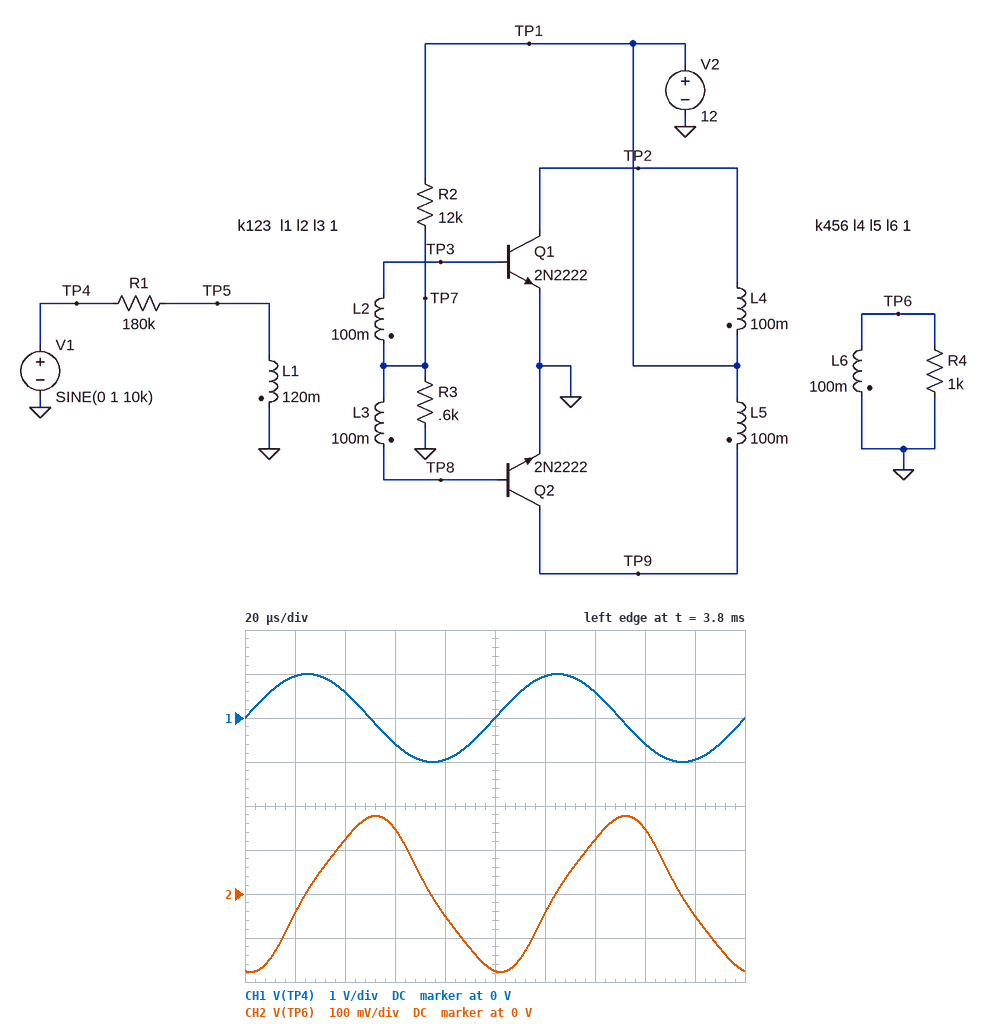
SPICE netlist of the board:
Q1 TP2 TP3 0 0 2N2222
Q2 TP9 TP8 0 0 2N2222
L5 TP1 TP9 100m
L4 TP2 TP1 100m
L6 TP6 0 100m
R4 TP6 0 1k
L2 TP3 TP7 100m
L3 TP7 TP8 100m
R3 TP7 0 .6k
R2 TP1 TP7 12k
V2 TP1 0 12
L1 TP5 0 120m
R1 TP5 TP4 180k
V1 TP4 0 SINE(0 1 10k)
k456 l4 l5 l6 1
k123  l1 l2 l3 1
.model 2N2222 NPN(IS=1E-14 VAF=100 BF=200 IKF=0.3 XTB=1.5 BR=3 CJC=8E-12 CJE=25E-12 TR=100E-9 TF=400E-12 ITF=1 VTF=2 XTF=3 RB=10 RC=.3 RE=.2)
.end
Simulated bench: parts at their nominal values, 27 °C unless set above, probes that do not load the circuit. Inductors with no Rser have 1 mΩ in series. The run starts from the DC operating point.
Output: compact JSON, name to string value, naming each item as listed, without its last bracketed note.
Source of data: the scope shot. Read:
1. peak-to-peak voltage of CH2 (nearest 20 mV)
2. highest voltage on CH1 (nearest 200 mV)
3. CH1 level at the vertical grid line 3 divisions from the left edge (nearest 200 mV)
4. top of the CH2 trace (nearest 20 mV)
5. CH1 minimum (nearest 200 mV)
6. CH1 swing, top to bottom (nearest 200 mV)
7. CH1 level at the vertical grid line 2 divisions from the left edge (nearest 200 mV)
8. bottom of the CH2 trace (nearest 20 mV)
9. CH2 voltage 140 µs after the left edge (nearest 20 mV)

{"peak-to-peak voltage of CH2": "360 mV", "highest voltage on CH1": "1.0 V", "CH1 level at the vertical grid line 3 divisions from the left edge": "-600 mV", "top of the CH2 trace": "180 mV", "CH1 minimum": "-1.0 V", "CH1 swing, top to bottom": "2.0 V", "CH1 level at the vertical grid line 2 divisions from the left edge": "600 mV", "bottom of the CH2 trace": "-180 mV", "CH2 voltage 140 µs after the left edge": "120 mV"}
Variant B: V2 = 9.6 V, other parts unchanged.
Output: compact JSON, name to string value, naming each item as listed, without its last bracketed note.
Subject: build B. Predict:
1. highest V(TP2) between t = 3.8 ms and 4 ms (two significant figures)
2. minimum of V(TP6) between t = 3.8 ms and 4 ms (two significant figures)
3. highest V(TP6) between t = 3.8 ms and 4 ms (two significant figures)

{"highest V(TP2) between t = 3.8 ms and 4 ms": "9.6 V", "minimum of V(TP6) between t = 3.8 ms and 4 ms": "-2.2 mV", "highest V(TP6) between t = 3.8 ms and 4 ms": "2.2 mV"}
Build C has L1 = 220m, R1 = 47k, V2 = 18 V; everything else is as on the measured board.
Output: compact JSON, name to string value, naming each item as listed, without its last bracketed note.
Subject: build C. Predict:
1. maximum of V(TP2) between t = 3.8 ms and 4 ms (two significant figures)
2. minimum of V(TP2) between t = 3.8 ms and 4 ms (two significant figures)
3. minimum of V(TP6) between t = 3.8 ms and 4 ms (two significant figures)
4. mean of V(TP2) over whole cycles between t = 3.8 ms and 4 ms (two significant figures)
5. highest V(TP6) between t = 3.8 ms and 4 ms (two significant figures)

{"maximum of V(TP2) between t = 3.8 ms and 4 ms": "23 V", "minimum of V(TP2) between t = 3.8 ms and 4 ms": "13 V", "minimum of V(TP6) between t = 3.8 ms and 4 ms": "-4.7 V", "mean of V(TP2) over whole cycles between t = 3.8 ms and 4 ms": "18 V", "highest V(TP6) between t = 3.8 ms and 4 ms": "4.7 V"}
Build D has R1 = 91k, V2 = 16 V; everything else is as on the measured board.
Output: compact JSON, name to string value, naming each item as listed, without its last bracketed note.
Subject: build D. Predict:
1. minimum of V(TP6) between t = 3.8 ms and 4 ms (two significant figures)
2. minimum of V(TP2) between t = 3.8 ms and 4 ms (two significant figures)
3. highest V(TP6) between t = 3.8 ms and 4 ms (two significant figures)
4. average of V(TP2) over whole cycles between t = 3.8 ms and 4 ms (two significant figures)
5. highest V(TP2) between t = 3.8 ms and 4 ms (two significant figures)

{"minimum of V(TP6) between t = 3.8 ms and 4 ms": "-2.2 V", "minimum of V(TP2) between t = 3.8 ms and 4 ms": "14 V", "highest V(TP6) between t = 3.8 ms and 4 ms": "2.2 V", "average of V(TP2) over whole cycles between t = 3.8 ms and 4 ms": "16 V", "highest V(TP2) between t = 3.8 ms and 4 ms": "18 V"}
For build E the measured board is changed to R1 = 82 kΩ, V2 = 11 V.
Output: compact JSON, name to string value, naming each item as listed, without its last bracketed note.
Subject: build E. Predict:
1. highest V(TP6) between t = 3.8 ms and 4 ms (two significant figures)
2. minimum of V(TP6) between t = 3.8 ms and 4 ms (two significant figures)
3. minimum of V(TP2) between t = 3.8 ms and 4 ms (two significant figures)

{"highest V(TP6) between t = 3.8 ms and 4 ms": "170 mV", "minimum of V(TP6) between t = 3.8 ms and 4 ms": "-170 mV", "minimum of V(TP2) between t = 3.8 ms and 4 ms": "11 V"}
